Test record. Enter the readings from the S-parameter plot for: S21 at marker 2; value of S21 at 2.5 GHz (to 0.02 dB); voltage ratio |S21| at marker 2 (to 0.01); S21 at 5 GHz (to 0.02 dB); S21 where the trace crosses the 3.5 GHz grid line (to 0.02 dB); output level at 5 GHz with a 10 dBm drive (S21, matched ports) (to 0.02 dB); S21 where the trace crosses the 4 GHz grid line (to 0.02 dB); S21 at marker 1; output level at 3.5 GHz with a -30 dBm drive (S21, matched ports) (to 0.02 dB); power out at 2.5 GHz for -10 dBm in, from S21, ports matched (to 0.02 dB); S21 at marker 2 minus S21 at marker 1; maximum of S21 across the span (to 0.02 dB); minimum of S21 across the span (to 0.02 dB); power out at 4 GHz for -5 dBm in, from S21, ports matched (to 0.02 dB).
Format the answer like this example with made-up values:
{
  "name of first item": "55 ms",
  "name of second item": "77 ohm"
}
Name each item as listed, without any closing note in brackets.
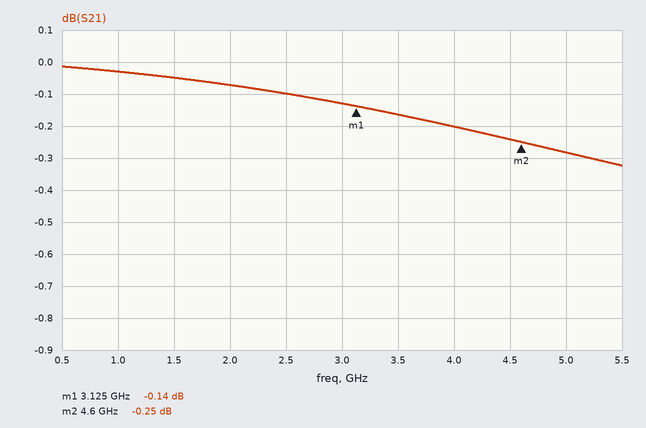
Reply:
{
  "S21 at marker 2": "-0.25 dB",
  "value of S21 at 2.5 GHz": "-0.10 dB",
  "voltage ratio |S21| at marker 2": "0.97",
  "S21 at 5 GHz": "-0.28 dB",
  "S21 where the trace crosses the 3.5 GHz grid line": "-0.16 dB",
  "output level at 5 GHz with a 10 dBm drive (S21, matched ports)": "9.72 dBm",
  "S21 where the trace crosses the 4 GHz grid line": "-0.20 dB",
  "S21 at marker 1": "-0.14 dB",
  "output level at 3.5 GHz with a -30 dBm drive (S21, matched ports)": "-30.16 dBm",
  "power out at 2.5 GHz for -10 dBm in, from S21, ports matched": "-10.10 dBm",
  "S21 at marker 2 minus S21 at marker 1": "-0.11 dB",
  "maximum of S21 across the span": "-0.02 dB",
  "minimum of S21 across the span": "-0.32 dB",
  "power out at 4 GHz for -5 dBm in, from S21, ports matched": "-5.20 dBm"
}
